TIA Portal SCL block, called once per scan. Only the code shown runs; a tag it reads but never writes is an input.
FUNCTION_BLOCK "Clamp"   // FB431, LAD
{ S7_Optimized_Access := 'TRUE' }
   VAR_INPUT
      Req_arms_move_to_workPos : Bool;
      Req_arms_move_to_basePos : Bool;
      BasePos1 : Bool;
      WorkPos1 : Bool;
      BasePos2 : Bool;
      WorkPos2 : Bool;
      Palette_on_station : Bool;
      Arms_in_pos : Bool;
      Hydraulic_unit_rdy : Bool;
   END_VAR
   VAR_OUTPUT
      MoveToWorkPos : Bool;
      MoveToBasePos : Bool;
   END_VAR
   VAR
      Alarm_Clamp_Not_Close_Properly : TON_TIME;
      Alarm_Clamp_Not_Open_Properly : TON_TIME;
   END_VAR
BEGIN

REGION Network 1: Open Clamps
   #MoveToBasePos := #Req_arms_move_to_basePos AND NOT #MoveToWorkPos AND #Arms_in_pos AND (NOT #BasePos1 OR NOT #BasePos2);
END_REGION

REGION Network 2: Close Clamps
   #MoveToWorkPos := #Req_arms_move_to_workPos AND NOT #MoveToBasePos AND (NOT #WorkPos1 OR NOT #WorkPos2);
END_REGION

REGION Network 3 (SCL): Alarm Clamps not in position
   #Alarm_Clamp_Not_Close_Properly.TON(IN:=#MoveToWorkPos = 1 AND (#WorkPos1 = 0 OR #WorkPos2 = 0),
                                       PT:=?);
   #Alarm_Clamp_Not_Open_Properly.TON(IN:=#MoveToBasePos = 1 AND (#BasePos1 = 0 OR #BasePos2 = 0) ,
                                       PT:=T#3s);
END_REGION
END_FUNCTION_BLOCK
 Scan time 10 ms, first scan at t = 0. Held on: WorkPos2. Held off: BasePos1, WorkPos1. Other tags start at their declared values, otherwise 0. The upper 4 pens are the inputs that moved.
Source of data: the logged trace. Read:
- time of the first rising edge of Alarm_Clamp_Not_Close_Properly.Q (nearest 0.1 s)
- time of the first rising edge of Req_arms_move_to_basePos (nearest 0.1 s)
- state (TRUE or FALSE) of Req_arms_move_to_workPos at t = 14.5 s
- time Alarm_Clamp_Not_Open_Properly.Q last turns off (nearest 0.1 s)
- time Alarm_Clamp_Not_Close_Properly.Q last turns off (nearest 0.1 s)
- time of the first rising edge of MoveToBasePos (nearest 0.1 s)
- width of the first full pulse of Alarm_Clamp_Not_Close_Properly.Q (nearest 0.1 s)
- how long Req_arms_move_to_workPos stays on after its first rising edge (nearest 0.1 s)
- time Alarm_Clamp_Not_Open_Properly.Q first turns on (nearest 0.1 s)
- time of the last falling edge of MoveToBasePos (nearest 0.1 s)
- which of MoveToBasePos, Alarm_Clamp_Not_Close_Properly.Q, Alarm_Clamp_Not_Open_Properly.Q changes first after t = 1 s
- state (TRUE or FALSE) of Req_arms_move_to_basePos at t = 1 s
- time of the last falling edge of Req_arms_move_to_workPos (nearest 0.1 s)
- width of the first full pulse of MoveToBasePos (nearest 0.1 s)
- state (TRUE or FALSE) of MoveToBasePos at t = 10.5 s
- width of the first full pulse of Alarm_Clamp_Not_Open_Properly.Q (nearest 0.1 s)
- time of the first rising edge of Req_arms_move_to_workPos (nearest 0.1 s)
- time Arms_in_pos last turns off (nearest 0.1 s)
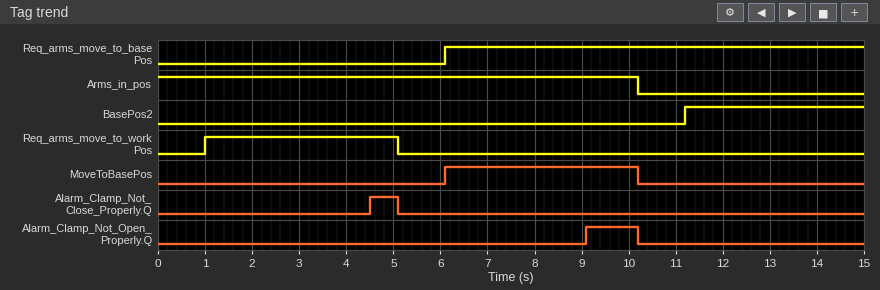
4.5 s
6.1 s
FALSE
10.2 s
5.1 s
6.1 s
0.6 s
4.1 s
9.1 s
10.2 s
Alarm_Clamp_Not_Close_Properly.Q
FALSE
5.1 s
4.1 s
FALSE
1.1 s
1.0 s
10.2 s
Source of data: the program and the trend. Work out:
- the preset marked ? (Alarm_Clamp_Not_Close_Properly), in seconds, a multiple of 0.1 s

3.5 s
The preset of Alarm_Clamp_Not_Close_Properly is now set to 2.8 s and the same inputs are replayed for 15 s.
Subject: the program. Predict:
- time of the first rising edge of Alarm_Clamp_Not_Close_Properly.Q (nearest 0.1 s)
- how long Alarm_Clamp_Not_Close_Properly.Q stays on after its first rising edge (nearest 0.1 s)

3.8 s
1.3 s
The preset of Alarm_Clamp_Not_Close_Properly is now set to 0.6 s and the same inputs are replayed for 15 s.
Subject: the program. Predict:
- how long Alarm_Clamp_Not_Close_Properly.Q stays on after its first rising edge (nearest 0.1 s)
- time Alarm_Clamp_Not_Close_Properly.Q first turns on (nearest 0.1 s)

3.5 s
1.6 s
